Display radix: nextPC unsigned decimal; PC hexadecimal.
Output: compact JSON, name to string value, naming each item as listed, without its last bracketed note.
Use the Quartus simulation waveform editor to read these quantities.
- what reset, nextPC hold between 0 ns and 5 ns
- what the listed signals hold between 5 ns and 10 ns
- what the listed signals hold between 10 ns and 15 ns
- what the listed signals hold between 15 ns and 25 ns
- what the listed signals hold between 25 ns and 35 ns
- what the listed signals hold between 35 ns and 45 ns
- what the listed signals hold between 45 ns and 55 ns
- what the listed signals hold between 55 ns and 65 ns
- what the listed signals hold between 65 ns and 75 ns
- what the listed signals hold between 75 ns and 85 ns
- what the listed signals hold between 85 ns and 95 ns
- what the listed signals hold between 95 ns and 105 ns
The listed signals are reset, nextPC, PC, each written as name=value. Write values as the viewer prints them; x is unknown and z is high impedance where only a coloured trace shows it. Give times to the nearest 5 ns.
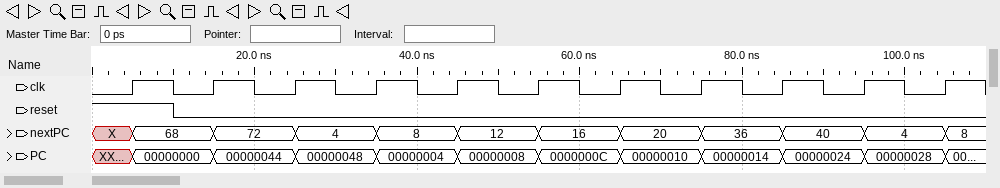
{"what reset, nextPC hold between 0 ns and 5 ns": "reset=1, nextPC=X", "what the listed signals hold between 5 ns and 10 ns": "reset=1, nextPC=68, PC=00000000", "what the listed signals hold between 10 ns and 15 ns": "reset=0, nextPC=68, PC=00000000", "what the listed signals hold between 15 ns and 25 ns": "reset=0, nextPC=72, PC=00000044", "what the listed signals hold between 25 ns and 35 ns": "reset=0, nextPC=4, PC=00000048", "what the listed signals hold between 35 ns and 45 ns": "reset=0, nextPC=8, PC=00000004", "what the listed signals hold between 45 ns and 55 ns": "reset=0, nextPC=12, PC=00000008", "what the listed signals hold between 55 ns and 65 ns": "reset=0, nextPC=16, PC=0000000C", "what the listed signals hold between 65 ns and 75 ns": "reset=0, nextPC=20, PC=00000010", "what the listed signals hold between 75 ns and 85 ns": "reset=0, nextPC=36, PC=00000014", "what the listed signals hold between 85 ns and 95 ns": "reset=0, nextPC=40, PC=00000024", "what the listed signals hold between 95 ns and 105 ns": "reset=0, nextPC=4, PC=00000028"}
